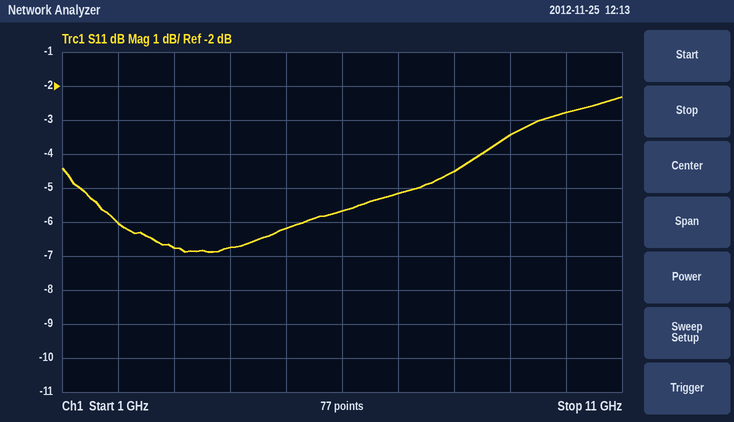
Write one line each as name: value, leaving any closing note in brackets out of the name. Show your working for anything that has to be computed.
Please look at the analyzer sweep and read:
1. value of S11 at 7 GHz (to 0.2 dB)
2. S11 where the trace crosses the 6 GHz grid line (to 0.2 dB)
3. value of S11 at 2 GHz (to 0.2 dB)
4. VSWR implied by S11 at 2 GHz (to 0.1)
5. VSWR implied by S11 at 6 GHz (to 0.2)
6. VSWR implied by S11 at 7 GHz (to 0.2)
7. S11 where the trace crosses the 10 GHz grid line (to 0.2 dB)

value of S11 at 7 GHz: -5.2 dB
S11 where the trace crosses the 6 GHz grid line: -5.6 dB
value of S11 at 2 GHz: -6.0 dB
VSWR implied by S11 at 2 GHz: |Γ| = 10^(-6/20) = 0.5012; VSWR = (1 + 0.5012)/(1 − 0.5012) ≈ 3.0
VSWR implied by S11 at 6 GHz: |Γ| = 10^(-5.6/20) = 0.5248; VSWR = (1 + 0.5248)/(1 − 0.5248) ≈ 3.2
VSWR implied by S11 at 7 GHz: |Γ| = 10^(-5.2/20) = 0.5495; VSWR = (1 + 0.5495)/(1 − 0.5495) ≈ 3.4
S11 where the trace crosses the 10 GHz grid line: -2.8 dB
